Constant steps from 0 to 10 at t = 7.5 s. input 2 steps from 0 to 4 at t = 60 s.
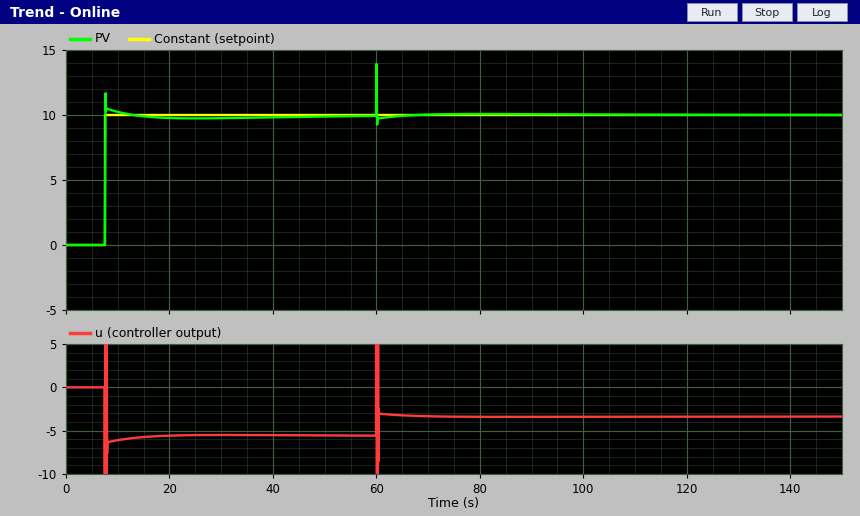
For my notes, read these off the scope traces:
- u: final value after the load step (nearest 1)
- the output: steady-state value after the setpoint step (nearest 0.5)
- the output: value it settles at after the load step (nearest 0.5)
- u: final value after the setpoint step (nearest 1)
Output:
-3
10.0
10.0
-6
